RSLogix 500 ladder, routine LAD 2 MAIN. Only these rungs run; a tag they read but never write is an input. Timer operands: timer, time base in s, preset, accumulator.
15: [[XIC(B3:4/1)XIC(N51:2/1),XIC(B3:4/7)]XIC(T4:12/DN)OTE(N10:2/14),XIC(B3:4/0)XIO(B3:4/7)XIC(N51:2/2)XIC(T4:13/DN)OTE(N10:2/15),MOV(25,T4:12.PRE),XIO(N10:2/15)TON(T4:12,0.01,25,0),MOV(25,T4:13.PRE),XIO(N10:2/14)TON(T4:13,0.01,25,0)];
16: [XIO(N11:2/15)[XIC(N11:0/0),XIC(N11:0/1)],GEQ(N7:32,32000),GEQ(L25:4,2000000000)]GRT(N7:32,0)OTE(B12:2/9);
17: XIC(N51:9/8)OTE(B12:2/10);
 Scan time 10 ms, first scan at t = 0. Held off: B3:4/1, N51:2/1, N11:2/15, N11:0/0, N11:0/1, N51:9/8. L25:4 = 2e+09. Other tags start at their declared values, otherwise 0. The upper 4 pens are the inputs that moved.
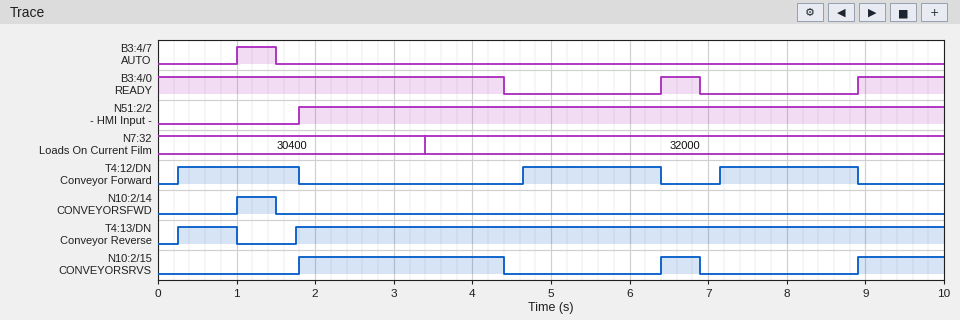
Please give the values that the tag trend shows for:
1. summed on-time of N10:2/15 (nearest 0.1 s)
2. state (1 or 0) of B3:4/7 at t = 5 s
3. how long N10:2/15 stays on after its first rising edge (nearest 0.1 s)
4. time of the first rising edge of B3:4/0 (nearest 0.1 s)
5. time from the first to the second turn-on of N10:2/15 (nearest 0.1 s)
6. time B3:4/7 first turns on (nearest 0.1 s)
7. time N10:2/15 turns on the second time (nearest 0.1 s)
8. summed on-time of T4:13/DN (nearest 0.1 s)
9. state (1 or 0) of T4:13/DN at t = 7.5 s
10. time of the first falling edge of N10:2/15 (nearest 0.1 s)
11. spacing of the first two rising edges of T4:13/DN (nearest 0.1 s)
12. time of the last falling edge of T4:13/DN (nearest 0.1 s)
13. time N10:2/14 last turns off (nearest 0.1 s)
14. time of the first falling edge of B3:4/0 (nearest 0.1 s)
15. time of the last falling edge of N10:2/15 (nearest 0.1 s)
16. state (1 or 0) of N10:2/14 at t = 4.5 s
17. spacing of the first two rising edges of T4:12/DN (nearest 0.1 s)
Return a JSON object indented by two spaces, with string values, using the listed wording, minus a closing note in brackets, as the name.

{
  "summed on-time of N10:2/15": "4.2 s",
  "state (1 or 0) of B3:4/7 at t = 5 s": "0",
  "how long N10:2/15 stays on after its first rising edge": "2.6 s",
  "time of the first rising edge of B3:4/0": "6.4 s",
  "time from the first to the second turn-on of N10:2/15": "4.6 s",
  "time B3:4/7 first turns on": "1.0 s",
  "time N10:2/15 turns on the second time": "6.4 s",
  "summed on-time of T4:13/DN": "9.0 s",
  "state (1 or 0) of T4:13/DN at t = 7.5 s": "1",
  "time of the first falling edge of N10:2/15": "4.4 s",
  "spacing of the first two rising edges of T4:13/DN": "1.5 s",
  "time of the last falling edge of T4:13/DN": "1.0 s",
  "time N10:2/14 last turns off": "1.5 s",
  "time of the first falling edge of B3:4/0": "4.4 s",
  "time of the last falling edge of N10:2/15": "6.9 s",
  "state (1 or 0) of N10:2/14 at t = 4.5 s": "0",
  "spacing of the first two rising edges of T4:12/DN": "4.4 s"
}
